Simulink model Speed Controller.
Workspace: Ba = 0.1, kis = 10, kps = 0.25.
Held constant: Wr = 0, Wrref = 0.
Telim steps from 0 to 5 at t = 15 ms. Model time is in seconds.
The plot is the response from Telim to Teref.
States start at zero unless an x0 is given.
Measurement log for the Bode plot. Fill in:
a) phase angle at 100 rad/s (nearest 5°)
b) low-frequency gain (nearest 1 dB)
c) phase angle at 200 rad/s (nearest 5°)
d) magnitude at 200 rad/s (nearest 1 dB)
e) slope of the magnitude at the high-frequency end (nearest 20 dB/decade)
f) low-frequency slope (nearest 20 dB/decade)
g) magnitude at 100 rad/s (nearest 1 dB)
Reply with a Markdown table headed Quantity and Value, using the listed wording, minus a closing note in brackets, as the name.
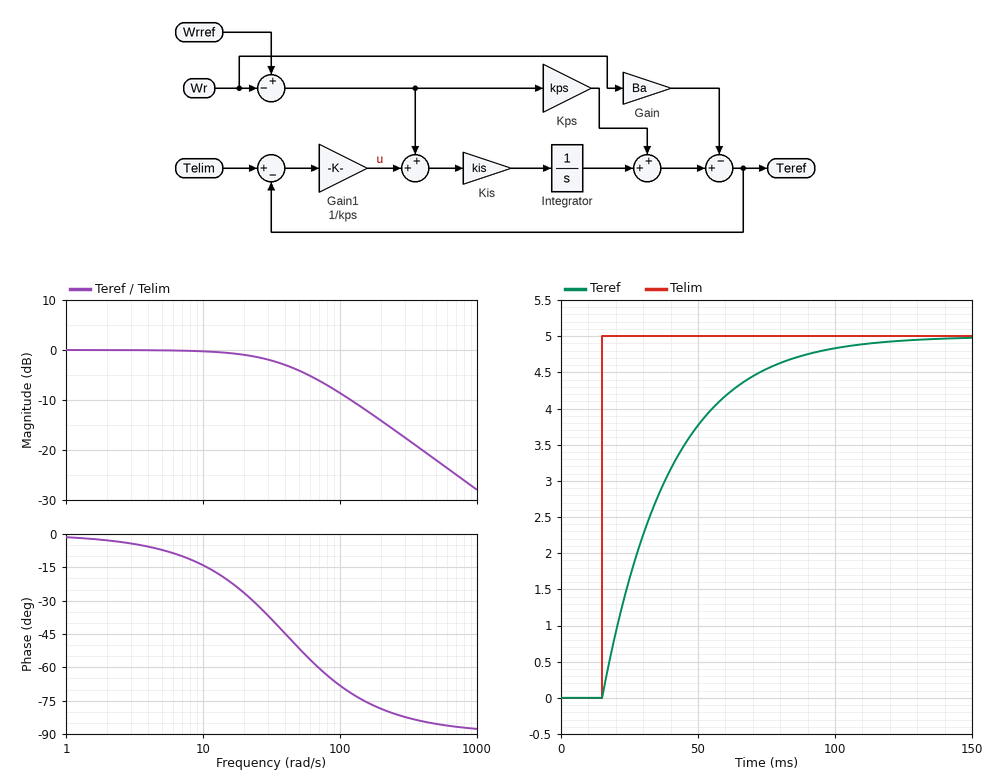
| Quantity | Value |
|---|---|
| phase angle at 100 rad/s | -70° |
| low-frequency gain | 0 dB |
| phase angle at 200 rad/s | -80° |
| magnitude at 200 rad/s | -14 dB |
| slope of the magnitude at the high-frequency end | -20 dB/decade |
| low-frequency slope | 0 dB/decade |
| magnitude at 100 rad/s | -9 dB |
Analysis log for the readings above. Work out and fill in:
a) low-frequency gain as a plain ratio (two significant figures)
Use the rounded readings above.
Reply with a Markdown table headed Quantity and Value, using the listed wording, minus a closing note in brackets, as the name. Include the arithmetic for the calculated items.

| Quantity | Value |
|---|---|
| low-frequency gain as a plain ratio | 10^(0 / 20) = 1.0 |
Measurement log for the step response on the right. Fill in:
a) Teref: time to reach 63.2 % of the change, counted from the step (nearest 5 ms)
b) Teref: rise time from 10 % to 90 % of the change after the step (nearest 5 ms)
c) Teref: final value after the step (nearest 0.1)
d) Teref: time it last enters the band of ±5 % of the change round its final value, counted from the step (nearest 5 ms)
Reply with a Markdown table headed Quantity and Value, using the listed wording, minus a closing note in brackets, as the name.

| Quantity | Value |
|---|---|
| Teref: time to reach 63.2 % of the change, counted from the step | 25 ms |
| Teref: rise time from 10 % to 90 % of the change after the step | 55 ms |
| Teref: final value after the step | 5.0 |
| Teref: time it last enters the band of ±5 % of the change round its final value, counted from the step | 75 ms |
